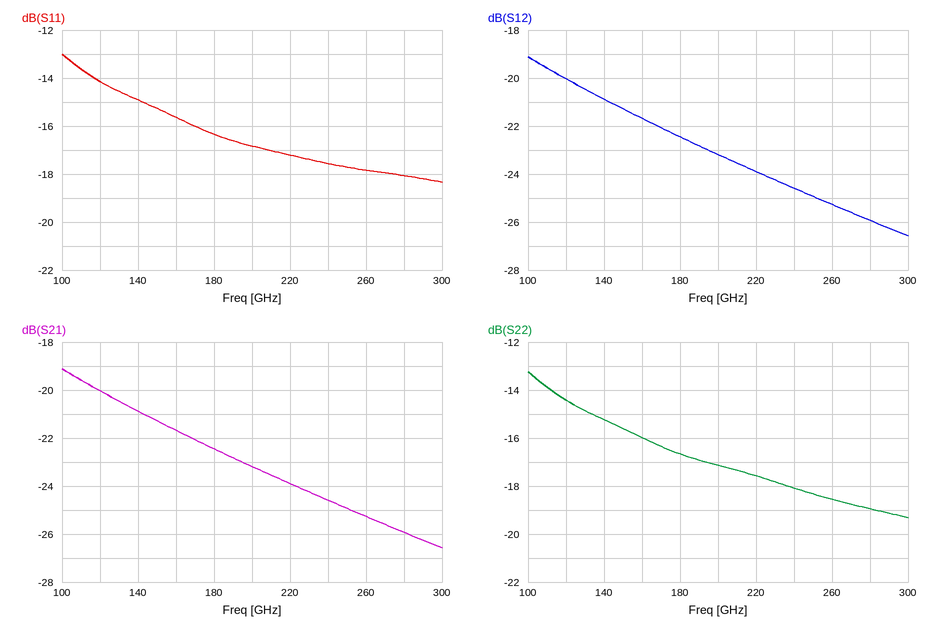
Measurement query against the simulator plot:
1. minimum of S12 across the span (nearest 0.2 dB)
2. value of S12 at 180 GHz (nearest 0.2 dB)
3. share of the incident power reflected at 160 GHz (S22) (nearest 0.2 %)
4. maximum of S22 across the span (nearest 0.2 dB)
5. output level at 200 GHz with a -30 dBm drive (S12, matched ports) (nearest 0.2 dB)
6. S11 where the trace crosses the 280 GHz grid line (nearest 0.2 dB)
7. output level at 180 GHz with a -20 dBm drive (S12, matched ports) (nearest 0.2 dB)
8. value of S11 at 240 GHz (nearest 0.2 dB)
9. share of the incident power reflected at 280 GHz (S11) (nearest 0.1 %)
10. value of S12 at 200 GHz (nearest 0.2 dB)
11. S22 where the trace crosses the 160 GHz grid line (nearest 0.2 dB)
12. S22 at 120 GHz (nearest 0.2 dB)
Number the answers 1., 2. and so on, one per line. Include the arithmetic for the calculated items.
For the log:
1. -26.6 dB
2. -22.4 dB
3. 10^(-16/10) ≈ 2.51 %, so 2.6 % to the nearest 0.2 %
4. -13.2 dB
5. -30 dBm + (-23.2 dB) = -53.2 dBm
6. -18.0 dB
7. -20 dBm + (-22.4 dB) = -42.4 dBm
8. -17.6 dB
9. 10^(-18/10) ≈ 1.6 %
10. -23.2 dB
11. -16.0 dB
12. -14.4 dB
